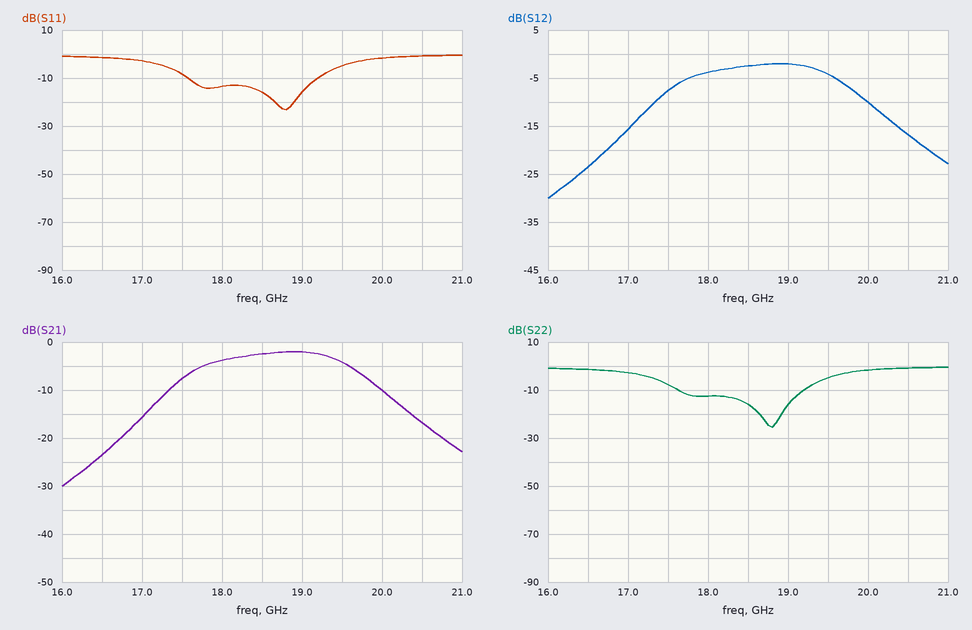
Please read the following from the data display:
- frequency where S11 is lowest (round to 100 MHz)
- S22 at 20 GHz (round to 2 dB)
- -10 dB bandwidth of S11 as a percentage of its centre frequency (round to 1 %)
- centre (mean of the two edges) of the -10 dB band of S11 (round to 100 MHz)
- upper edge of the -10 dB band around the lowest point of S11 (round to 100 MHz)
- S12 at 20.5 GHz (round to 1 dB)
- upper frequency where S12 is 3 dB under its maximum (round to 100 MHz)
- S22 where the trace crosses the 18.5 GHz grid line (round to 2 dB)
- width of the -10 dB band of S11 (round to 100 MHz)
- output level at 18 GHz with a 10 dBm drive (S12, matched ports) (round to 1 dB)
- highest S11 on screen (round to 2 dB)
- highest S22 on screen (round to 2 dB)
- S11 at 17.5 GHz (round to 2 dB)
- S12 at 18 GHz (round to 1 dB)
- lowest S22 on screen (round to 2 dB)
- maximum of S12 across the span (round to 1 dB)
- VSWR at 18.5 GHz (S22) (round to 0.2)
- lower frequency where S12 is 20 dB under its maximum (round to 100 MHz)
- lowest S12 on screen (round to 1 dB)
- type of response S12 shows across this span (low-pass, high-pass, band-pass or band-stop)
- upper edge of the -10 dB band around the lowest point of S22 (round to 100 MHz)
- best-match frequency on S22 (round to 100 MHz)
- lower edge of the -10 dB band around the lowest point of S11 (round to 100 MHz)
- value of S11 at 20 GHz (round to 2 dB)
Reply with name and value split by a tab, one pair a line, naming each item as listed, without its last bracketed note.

frequency where S11 is lowest	18.8 GHz
S22 at 20 GHz	-2 dB
-10 dB bandwidth of S11 as a percentage of its centre frequency	9 %
centre (mean of the two edges) of the -10 dB band of S11	18.4 GHz
upper edge of the -10 dB band around the lowest point of S11	19.2 GHz
S12 at 20.5 GHz	-17 dB
upper frequency where S12 is 3 dB under its maximum	19.6 GHz
S22 where the trace crosses the 18.5 GHz grid line	-16 dB
width of the -10 dB band of S11	1.6 GHz
output level at 18 GHz with a 10 dBm drive (S12, matched ports)	6 dBm
highest S11 on screen	0 dB
highest S22 on screen	0 dB
S11 at 17.5 GHz	-8 dB
S12 at 18 GHz	-4 dB
lowest S22 on screen	-26 dB
maximum of S12 across the span	-2 dB
VSWR at 18.5 GHz (S22)	1.4
lower frequency where S12 is 20 dB under its maximum	16.6 GHz
lowest S12 on screen	-30 dB
type of response S12 shows across this span	band-pass
upper edge of the -10 dB band around the lowest point of S22	19.2 GHz
best-match frequency on S22	18.8 GHz
lower edge of the -10 dB band around the lowest point of S11	17.6 GHz
value of S11 at 20 GHz	-2 dB
